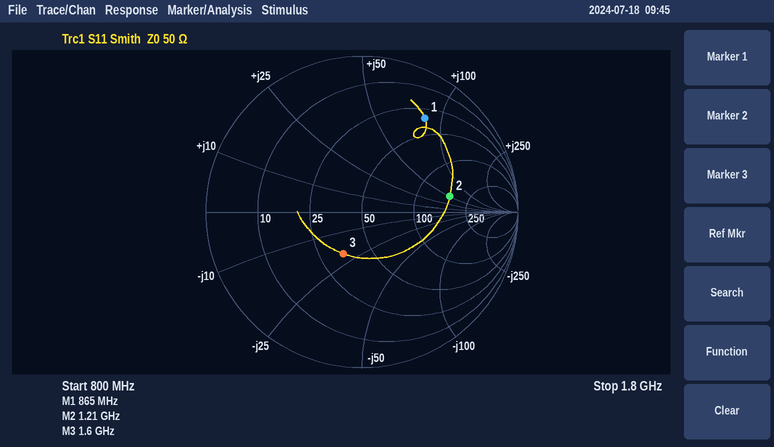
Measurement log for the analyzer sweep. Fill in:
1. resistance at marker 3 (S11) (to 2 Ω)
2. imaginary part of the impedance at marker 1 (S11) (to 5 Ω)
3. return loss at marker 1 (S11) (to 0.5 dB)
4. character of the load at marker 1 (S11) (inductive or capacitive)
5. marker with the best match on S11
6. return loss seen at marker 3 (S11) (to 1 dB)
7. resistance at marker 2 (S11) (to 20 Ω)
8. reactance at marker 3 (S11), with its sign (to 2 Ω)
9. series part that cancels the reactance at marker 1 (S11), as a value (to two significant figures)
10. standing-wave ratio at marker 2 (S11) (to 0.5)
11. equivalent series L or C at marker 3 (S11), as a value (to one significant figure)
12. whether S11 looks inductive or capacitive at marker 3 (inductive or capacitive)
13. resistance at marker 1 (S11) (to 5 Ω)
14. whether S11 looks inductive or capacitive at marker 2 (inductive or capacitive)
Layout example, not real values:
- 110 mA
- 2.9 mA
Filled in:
- 34 Ω
- +85 Ω
- 3.0 dB
- inductive
- marker 3
- 11 dB
- 160 Ω
- -20 Ω
- 2.2 pF
- 3.5
- 5 pF
- capacitive
- 35 Ω
- inductive
